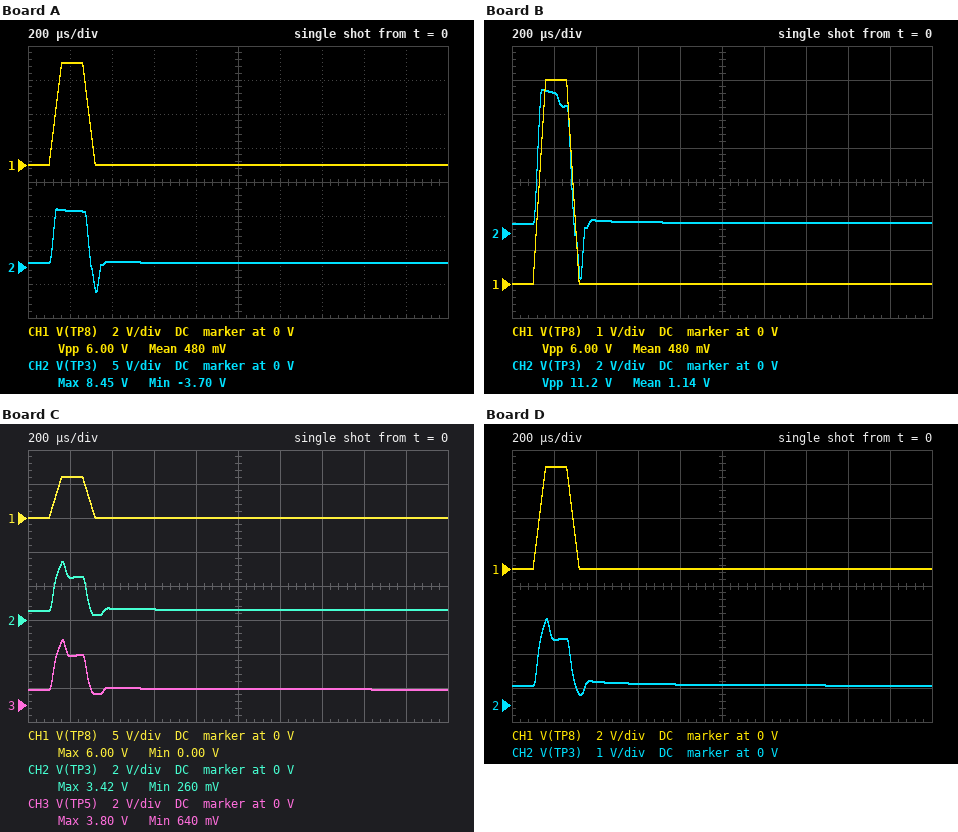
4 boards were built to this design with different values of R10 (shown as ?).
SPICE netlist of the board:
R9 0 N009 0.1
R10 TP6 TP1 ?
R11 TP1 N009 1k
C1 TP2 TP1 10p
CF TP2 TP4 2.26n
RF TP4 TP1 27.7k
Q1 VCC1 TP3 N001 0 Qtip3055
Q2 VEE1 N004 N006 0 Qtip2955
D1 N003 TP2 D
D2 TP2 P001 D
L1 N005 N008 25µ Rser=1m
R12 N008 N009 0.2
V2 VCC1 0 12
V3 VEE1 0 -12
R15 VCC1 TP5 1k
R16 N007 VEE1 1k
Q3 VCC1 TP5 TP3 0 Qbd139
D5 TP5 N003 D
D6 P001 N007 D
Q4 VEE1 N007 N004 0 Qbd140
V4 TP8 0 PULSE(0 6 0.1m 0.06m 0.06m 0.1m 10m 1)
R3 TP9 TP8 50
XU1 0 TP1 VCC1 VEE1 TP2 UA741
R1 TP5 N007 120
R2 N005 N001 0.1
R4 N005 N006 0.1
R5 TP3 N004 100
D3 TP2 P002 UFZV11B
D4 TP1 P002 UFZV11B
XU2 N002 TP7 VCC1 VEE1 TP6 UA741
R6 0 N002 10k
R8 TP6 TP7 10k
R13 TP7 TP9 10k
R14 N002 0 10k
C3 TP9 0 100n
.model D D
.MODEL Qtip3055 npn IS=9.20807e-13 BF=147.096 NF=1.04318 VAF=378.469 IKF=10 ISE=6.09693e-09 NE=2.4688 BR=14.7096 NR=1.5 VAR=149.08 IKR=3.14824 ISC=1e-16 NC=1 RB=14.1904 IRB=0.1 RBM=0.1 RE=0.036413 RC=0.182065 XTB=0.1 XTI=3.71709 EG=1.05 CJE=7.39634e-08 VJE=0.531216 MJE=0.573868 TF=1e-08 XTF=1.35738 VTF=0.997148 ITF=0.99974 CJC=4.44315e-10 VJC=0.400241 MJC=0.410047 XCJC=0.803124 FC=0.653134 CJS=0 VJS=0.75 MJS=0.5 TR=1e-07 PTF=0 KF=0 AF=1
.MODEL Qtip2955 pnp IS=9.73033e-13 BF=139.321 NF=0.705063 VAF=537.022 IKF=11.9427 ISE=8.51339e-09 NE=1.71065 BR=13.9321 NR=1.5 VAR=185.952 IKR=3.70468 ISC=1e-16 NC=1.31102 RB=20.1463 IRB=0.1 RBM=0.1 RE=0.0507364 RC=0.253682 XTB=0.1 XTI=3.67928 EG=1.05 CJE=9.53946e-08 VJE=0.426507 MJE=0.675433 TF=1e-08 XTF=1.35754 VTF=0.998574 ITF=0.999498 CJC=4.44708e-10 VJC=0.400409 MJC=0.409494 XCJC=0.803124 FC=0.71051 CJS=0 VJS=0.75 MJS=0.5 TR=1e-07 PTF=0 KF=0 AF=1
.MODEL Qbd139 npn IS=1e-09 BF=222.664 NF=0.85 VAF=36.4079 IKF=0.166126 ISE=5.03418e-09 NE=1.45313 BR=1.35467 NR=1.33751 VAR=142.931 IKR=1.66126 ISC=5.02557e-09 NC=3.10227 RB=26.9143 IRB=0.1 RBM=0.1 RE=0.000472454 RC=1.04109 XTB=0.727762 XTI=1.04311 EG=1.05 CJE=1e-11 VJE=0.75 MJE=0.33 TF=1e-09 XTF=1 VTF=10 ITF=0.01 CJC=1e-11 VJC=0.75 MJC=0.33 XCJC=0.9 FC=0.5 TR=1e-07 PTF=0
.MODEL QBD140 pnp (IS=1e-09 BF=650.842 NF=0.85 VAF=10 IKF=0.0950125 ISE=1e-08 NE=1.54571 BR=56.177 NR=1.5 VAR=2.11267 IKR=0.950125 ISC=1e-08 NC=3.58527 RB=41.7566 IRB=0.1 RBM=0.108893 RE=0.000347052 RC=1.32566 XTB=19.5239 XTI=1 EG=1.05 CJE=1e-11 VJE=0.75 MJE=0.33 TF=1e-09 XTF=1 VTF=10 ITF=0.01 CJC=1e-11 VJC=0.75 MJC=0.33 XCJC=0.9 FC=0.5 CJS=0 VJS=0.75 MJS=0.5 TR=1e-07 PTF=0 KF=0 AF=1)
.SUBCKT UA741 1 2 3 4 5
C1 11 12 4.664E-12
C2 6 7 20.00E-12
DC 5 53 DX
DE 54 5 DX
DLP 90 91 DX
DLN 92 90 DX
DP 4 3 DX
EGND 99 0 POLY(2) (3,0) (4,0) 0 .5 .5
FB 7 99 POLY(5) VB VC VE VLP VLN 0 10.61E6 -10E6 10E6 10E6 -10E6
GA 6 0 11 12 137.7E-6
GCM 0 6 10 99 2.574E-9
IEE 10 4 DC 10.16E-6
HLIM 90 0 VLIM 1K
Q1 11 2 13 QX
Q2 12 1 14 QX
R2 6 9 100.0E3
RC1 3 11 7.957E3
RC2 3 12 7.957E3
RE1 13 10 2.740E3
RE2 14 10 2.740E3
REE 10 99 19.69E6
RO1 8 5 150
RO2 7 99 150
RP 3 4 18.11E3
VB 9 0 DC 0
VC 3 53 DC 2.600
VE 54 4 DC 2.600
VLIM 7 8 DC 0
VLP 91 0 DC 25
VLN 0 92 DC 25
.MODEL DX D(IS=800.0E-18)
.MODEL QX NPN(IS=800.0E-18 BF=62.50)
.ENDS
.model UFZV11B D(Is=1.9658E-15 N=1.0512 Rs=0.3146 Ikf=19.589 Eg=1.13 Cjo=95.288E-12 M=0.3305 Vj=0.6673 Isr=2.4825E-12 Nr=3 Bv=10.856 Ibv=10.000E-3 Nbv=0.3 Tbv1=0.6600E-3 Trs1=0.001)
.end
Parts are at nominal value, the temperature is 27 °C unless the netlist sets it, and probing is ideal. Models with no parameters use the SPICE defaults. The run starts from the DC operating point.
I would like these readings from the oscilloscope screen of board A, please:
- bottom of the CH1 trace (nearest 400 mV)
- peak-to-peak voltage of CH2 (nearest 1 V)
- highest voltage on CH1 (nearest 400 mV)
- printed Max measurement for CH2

0 V
12 V
6.0 V
8.45 V
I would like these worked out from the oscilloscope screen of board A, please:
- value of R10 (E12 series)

3.9 kΩ
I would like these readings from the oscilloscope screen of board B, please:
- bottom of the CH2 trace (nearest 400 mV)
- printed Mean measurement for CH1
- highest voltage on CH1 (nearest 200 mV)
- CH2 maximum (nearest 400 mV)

-2.8 V
480 mV
6.0 V
8.4 V
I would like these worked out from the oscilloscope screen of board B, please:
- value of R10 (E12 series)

4.7 kΩ
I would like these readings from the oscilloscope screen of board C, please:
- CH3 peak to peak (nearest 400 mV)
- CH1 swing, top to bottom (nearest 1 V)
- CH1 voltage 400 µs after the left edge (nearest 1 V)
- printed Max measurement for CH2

3.2 V
6 V
0 V
3.42 V
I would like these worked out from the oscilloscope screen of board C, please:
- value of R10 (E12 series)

18 kΩ
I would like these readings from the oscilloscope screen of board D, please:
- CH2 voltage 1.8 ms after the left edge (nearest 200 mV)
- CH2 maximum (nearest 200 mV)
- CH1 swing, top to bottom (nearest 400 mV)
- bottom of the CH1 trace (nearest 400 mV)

600 mV
2.6 V
6.0 V
0 V
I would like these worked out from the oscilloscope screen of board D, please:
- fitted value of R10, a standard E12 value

27 kΩ
